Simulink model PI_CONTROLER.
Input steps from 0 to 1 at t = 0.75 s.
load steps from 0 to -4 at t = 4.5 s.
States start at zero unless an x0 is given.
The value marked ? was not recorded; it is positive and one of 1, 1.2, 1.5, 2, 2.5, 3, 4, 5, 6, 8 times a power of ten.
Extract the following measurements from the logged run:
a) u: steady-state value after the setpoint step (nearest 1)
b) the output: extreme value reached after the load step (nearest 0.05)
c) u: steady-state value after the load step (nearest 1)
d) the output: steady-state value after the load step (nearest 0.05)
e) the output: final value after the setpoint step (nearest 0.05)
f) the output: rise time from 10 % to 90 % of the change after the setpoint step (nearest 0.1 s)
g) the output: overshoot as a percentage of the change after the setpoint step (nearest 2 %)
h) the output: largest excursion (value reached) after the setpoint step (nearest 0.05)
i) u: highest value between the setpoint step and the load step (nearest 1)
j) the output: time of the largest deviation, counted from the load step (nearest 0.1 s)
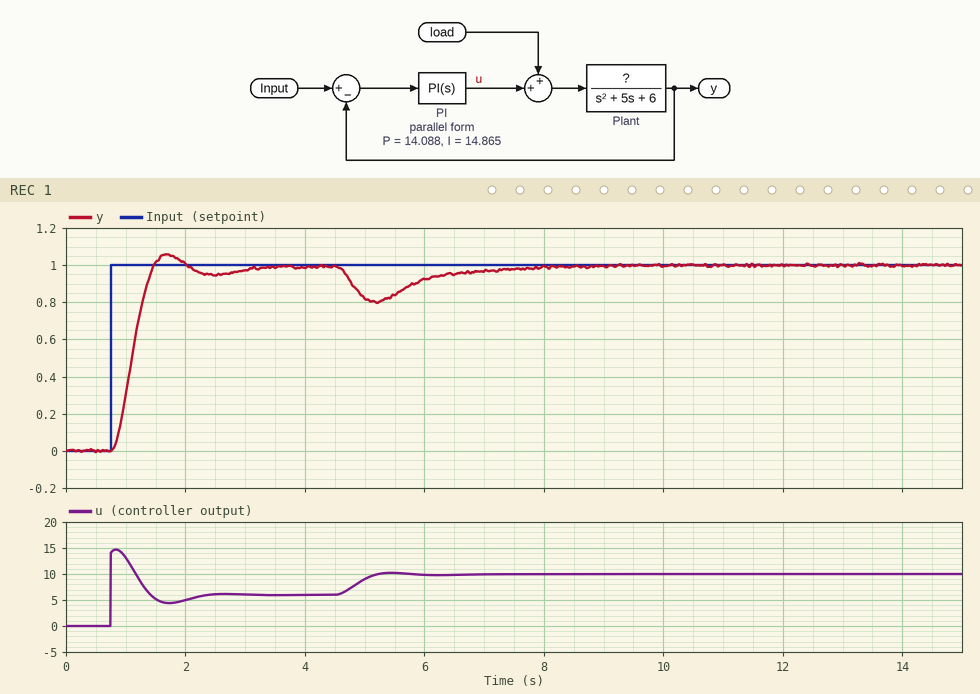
6
0.80
10
1.00
1.00
0.5 s
6 %
1.05
15
0.7 s
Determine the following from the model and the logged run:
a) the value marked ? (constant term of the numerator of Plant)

1
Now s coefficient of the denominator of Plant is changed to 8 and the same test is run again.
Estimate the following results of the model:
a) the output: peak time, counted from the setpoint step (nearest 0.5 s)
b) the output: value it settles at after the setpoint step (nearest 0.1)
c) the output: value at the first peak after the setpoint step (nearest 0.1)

1.5 s
1.0
1.0
